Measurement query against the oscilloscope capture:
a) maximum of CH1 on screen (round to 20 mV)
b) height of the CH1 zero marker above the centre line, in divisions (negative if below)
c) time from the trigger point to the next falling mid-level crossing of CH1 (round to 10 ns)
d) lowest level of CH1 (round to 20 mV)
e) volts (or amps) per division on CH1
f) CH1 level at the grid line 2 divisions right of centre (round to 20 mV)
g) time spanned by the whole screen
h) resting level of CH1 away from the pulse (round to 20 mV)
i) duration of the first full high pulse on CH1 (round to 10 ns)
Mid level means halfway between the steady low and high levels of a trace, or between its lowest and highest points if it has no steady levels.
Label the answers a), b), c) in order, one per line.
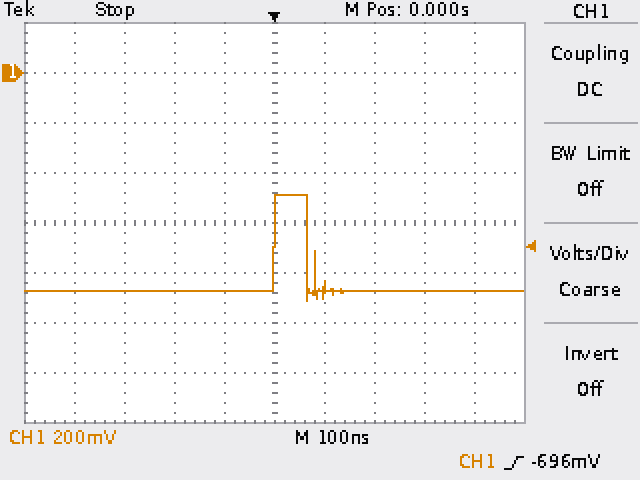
a) -480 mV
b) +3.0 div
c) 70 ns
d) -920 mV
e) 200 mV
f) -880 mV
g) 1 µs
h) -880 mV
i) 70 ns
